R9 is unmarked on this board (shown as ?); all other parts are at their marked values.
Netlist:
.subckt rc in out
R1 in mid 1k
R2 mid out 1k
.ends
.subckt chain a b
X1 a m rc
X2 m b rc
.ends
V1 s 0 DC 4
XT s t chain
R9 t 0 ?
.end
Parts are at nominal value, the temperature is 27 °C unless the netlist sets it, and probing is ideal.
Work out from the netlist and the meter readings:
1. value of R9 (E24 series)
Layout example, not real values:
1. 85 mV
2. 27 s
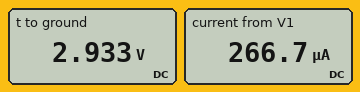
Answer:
1. 11 kΩ
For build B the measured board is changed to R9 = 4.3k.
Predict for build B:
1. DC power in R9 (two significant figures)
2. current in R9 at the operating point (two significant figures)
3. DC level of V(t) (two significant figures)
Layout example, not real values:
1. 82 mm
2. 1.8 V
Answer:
1. 1.0 mW
2. 480 µA
3. 2.1 V
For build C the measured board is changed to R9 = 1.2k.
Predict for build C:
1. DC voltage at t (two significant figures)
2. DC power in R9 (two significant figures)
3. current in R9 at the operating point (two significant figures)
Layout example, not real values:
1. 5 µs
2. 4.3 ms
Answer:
1. 920 mV
2. 710 µW
3. 770 µA
